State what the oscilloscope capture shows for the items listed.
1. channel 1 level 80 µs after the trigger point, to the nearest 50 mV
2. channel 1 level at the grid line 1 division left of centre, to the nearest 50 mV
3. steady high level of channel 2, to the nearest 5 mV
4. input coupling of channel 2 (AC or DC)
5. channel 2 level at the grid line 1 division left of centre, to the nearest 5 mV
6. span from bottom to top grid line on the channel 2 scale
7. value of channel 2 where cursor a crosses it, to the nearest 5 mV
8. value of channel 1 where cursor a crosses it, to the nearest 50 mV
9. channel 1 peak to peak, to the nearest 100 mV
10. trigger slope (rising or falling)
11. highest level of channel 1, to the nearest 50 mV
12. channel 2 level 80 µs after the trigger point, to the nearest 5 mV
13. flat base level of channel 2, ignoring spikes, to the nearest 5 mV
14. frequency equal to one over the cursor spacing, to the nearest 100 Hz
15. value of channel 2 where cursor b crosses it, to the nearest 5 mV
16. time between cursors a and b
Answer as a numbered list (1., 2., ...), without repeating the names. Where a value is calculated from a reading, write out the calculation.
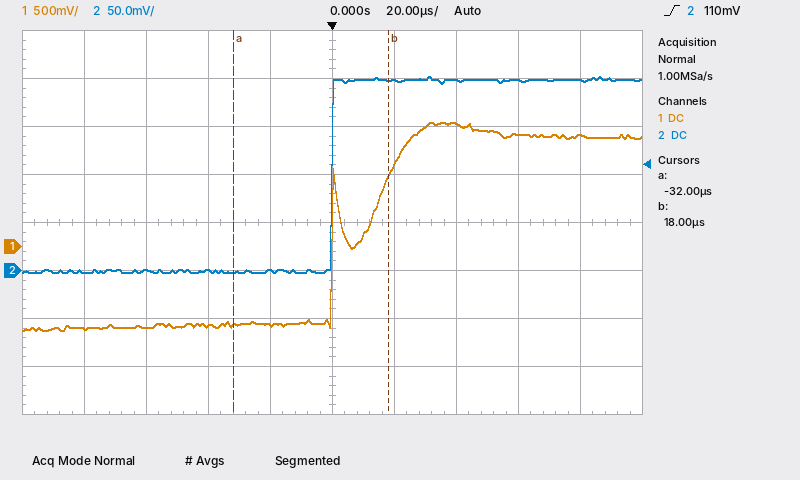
1. 1.15 V
2. -800 mV
3. 200 mV
4. DC
5. 0 mV
6. 400 mV
7. 0 mV
8. -800 mV
9. 2.20 V
10. rising
11. 1.30 V
12. 200 mV
13. 0 mV
14. 1 / 50 µs ≈ 20.0 kHz
15. 200 mV
16. 18 µs − (-32 µs) = 50 µs
